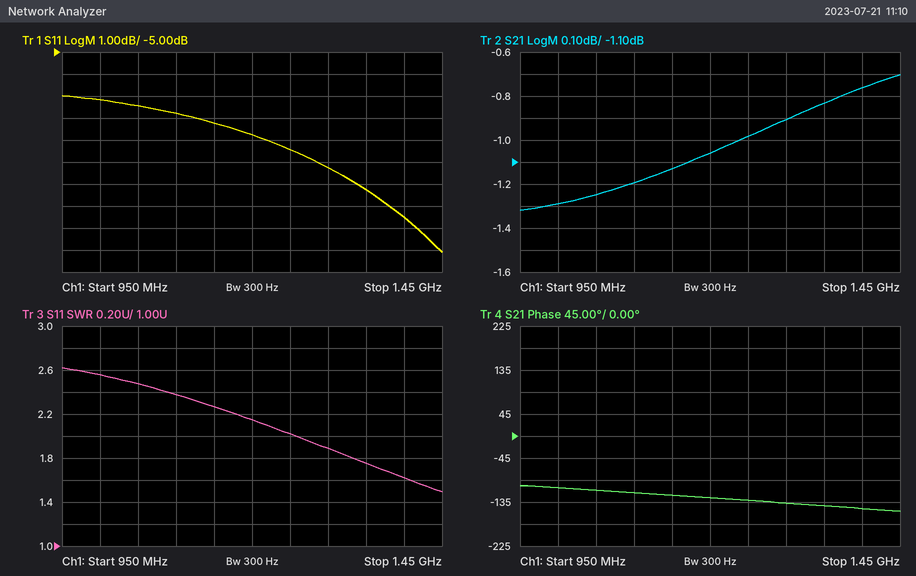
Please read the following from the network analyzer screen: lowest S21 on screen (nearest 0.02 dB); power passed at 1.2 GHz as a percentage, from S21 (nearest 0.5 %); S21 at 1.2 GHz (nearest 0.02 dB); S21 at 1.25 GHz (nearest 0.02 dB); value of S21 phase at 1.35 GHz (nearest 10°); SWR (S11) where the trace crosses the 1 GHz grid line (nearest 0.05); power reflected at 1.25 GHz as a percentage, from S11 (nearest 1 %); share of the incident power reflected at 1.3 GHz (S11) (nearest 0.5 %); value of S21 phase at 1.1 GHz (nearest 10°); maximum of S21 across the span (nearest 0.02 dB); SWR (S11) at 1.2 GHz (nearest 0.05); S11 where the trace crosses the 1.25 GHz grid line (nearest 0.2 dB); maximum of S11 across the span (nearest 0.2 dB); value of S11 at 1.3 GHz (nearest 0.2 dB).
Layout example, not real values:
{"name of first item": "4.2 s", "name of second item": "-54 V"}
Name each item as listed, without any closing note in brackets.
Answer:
{"lowest S21 on screen": "-1.32 dB", "power passed at 1.2 GHz as a percentage, from S21": "78.5 %", "S21 at 1.2 GHz": "-1.06 dB", "S21 at 1.25 GHz": "-0.98 dB", "value of S21 phase at 1.35 GHz": "-140°", "SWR (S11) where the trace crosses the 1 GHz grid line": "2.55", "power reflected at 1.25 GHz as a percentage, from S11": "11 %", "share of the incident power reflected at 1.3 GHz (S11)": "9.5 %", "value of S21 phase at 1.1 GHz": "-120°", "maximum of S21 across the span": "-0.70 dB", "SWR (S11) at 1.2 GHz": "2.15", "S11 where the trace crosses the 1.25 GHz grid line": "-9.4 dB", "maximum of S11 across the span": "-7.0 dB", "value of S11 at 1.3 GHz": "-10.2 dB"}
